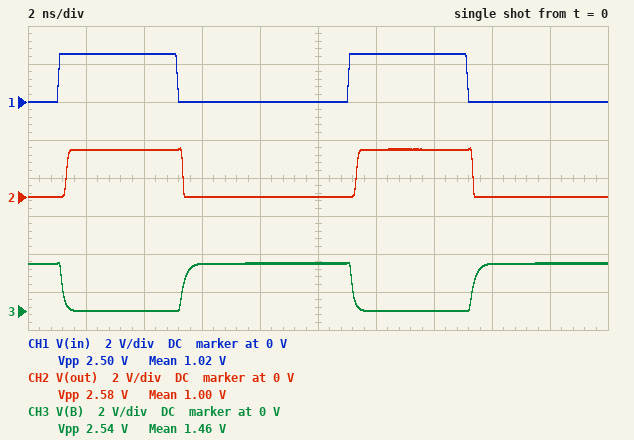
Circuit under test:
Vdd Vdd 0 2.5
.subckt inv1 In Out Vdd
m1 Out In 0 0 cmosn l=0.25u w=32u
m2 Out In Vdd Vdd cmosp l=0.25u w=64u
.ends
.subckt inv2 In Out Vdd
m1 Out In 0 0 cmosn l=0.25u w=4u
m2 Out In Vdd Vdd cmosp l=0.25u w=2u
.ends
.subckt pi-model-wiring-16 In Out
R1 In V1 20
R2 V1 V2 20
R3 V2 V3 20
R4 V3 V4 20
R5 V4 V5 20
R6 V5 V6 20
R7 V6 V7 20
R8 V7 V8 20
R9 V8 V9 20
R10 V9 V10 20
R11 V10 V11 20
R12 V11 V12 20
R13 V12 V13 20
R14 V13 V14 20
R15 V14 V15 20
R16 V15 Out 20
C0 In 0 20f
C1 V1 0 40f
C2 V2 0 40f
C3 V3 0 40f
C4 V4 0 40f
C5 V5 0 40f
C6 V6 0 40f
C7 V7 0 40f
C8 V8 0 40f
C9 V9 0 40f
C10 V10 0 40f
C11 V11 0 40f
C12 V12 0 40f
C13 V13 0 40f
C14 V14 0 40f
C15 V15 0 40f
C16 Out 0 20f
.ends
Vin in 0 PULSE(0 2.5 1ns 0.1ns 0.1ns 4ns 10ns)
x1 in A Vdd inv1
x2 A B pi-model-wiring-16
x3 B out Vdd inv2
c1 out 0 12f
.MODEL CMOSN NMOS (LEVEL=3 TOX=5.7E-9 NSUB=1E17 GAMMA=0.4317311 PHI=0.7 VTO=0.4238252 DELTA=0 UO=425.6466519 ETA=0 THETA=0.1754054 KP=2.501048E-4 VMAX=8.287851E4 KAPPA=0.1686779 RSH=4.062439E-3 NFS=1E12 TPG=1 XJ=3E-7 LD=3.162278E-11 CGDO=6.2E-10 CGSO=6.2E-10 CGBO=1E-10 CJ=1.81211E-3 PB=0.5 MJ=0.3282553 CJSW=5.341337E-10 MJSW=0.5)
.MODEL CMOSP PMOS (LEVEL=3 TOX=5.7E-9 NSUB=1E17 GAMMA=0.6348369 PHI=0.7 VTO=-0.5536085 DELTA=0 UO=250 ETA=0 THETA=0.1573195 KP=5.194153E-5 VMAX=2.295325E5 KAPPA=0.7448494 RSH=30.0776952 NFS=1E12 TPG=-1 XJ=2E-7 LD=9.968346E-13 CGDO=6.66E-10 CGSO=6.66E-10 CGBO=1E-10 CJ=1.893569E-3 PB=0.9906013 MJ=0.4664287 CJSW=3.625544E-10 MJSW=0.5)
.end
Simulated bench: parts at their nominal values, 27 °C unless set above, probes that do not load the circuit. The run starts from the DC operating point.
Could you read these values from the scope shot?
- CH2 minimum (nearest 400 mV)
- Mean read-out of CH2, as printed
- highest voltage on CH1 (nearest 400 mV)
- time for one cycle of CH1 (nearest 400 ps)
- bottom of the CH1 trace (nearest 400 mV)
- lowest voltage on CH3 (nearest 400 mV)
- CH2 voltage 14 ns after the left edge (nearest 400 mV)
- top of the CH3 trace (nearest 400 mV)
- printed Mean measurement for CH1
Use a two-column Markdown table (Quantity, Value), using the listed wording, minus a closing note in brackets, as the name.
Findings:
| Quantity | Value |
|---|---|
| CH2 minimum | 0 V |
| Mean read-out of CH2, as printed | 1.00 V |
| highest voltage on CH1 | 2.4 V |
| time for one cycle of CH1 | 10.0 ns |
| bottom of the CH1 trace | 0 V |
| lowest voltage on CH3 | 0 V |
| CH2 voltage 14 ns after the left edge | 2.4 V |
| top of the CH3 trace | 2.4 V |
| printed Mean measurement for CH1 | 1.02 V |
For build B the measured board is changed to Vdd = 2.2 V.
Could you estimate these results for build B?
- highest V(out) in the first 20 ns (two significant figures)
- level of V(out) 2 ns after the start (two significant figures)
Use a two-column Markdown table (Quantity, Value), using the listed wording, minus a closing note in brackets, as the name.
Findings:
| Quantity | Value |
|---|---|
| highest V(out) in the first 20 ns | 2.3 V |
| level of V(out) 2 ns after the start | 2.2 V |
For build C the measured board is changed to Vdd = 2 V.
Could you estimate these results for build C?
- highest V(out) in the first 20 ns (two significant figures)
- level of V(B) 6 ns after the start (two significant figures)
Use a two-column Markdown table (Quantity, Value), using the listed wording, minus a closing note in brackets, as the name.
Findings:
| Quantity | Value |
|---|---|
| highest V(out) in the first 20 ns | 2.1 V |
| level of V(B) 6 ns after the start | 2.0 V |
